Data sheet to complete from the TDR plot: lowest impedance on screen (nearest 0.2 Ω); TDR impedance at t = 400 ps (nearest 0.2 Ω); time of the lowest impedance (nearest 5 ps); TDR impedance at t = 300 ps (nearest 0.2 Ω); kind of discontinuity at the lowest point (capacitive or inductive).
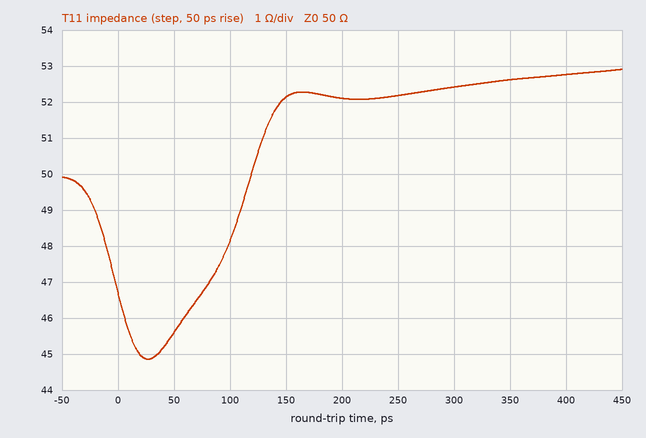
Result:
44.8 Ω
52.8 Ω
25 ps
52.4 Ω
capacitive
